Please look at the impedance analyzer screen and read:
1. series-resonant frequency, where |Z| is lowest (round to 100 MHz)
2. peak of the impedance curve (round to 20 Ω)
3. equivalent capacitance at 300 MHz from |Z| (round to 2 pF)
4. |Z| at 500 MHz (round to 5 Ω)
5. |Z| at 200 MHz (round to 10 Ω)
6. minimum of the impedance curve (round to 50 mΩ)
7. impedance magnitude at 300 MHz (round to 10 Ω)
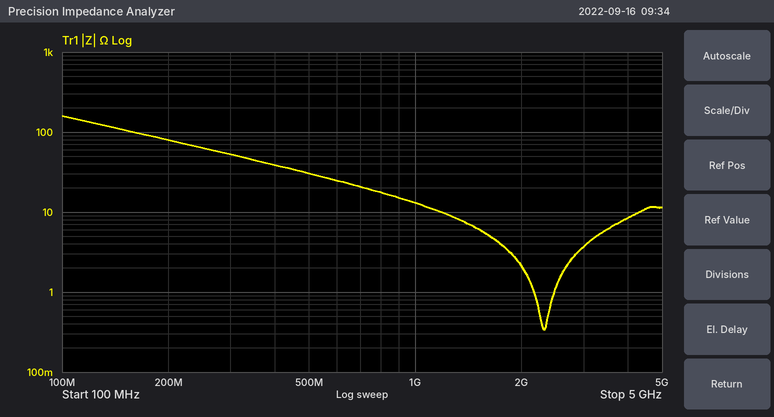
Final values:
2.3 GHz
160 Ω
10 pF
30 Ω
80 Ω
350 mΩ
50 Ω
